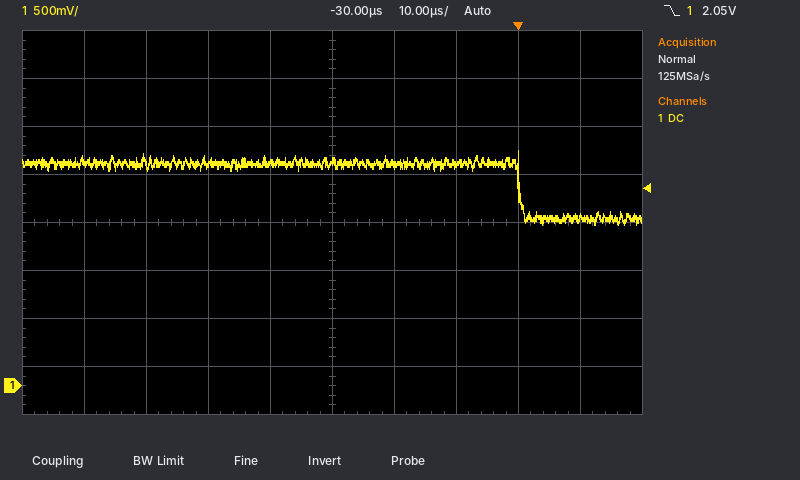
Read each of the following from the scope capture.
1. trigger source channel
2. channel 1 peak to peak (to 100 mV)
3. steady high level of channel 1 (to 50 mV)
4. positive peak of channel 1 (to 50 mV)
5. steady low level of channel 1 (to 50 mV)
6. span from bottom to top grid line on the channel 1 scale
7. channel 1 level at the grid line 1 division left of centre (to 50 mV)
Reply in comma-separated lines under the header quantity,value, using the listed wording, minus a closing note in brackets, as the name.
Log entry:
quantity,value
trigger source channel,channel 1
channel 1 peak to peak,800 mV
steady high level of channel 1,2.30 V
positive peak of channel 1,2.45 V
steady low level of channel 1,1.75 V
span from bottom to top grid line on the channel 1 scale,4 V
channel 1 level at the grid line 1 division left of centre,2.30 V
